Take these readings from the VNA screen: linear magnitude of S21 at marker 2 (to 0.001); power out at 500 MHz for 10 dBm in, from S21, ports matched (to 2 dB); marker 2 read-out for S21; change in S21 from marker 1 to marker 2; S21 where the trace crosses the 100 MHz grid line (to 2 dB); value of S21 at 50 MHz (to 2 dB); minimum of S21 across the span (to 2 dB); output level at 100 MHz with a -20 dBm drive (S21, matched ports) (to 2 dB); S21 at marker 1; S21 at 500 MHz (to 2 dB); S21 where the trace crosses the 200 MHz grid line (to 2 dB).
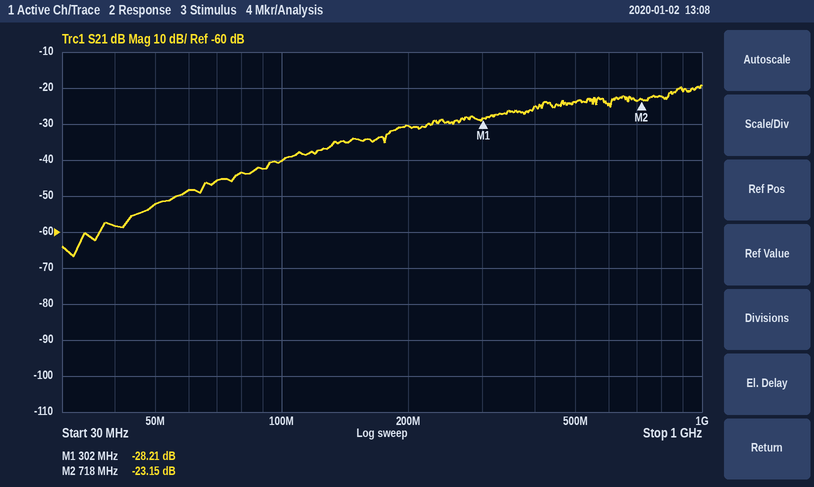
0.070
-14 dBm
-23.15 dB
5.06 dB
-40 dB
-52 dB
-66 dB
-60 dBm
-28.21 dB
-24 dB
-30 dB
